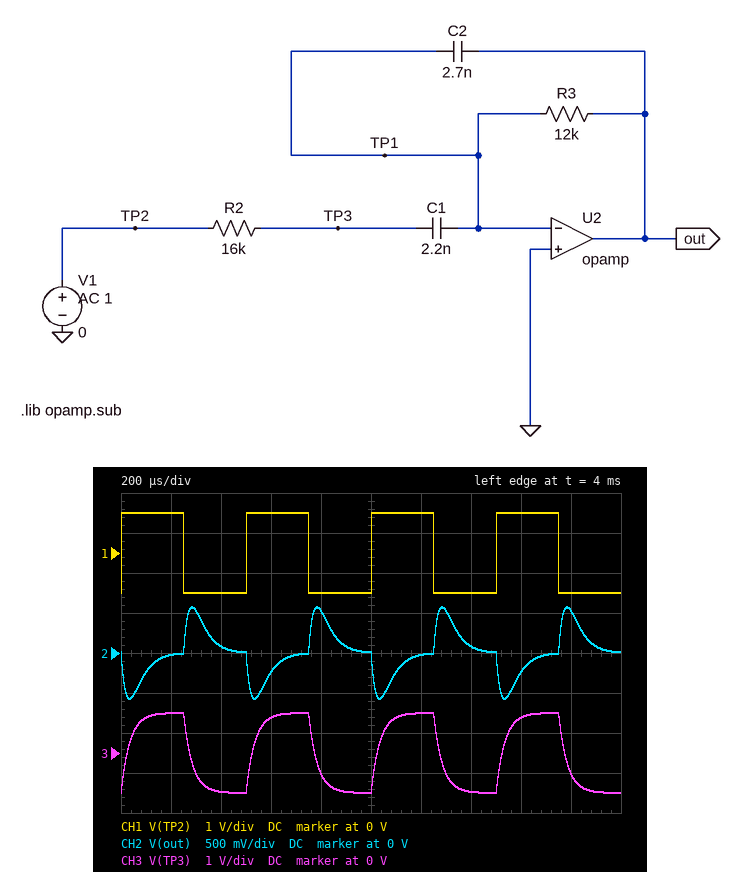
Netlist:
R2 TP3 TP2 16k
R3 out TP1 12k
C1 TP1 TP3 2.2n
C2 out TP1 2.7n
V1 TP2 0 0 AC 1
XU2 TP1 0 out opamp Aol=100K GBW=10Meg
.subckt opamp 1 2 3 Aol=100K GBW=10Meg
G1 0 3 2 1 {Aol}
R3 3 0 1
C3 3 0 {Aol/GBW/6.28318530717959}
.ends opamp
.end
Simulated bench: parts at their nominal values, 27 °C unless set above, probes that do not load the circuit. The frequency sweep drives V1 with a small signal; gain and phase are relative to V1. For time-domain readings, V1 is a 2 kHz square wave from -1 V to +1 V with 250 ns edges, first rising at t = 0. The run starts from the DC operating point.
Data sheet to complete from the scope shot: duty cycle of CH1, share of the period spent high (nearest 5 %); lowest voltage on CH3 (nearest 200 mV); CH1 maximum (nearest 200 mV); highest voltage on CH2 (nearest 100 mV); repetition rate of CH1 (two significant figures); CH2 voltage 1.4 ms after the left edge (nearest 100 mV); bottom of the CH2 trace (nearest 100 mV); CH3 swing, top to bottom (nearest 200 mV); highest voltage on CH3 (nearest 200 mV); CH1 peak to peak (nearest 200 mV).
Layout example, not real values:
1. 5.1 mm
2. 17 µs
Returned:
1. 50 %
2. -1.0 V
3. 1.0 V
4. 600 mV
5. 2.0 kHz
6. 100 mV
7. -600 mV
8. 2.0 V
9. 1.0 V
10. 2.0 V
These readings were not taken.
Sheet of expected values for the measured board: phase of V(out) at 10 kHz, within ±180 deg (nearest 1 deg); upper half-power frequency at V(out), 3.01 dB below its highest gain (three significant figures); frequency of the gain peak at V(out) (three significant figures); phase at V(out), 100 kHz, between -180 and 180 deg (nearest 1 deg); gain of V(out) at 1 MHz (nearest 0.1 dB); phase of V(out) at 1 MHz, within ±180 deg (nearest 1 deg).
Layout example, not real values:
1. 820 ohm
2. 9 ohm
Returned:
1. 140 deg
2. 11.4 kHz
3. 4.71 kHz
4. 95 deg
5. -48.7 dB
6. 85 deg
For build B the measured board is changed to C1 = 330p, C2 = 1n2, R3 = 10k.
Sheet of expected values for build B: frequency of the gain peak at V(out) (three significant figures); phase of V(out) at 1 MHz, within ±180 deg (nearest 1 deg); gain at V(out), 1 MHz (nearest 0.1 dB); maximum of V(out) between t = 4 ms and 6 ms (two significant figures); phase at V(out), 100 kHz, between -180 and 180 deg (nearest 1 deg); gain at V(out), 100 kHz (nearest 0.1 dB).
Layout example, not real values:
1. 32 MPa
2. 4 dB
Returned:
1. 20.0 kHz
2. 87 deg
3. -41.7 dB
4. 290 mV
5. 114 deg
6. -22.1 dB
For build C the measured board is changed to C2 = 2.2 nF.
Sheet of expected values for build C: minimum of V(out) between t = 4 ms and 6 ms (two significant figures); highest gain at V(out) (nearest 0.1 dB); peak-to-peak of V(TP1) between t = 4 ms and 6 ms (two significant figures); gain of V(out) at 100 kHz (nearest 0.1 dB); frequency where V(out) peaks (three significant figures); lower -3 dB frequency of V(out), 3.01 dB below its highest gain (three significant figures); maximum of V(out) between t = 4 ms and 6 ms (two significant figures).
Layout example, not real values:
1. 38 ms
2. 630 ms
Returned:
1. -630 mV
2. -7.4 dB
3. 1.8 mV
4. -26.9 dB
5. 5.22 kHz
6. 2.15 kHz
7. 630 mV
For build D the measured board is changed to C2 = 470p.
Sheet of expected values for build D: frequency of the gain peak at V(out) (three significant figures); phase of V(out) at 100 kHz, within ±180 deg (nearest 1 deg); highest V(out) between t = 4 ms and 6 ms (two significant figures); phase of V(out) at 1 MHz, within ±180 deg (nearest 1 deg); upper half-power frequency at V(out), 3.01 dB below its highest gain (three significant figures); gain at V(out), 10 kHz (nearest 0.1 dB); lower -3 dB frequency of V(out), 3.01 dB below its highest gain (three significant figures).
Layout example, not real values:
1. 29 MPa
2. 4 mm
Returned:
1. 11.3 kHz
2. 108 deg
3. 1.1 V
4. 86 deg
5. 36.2 kHz
6. -3.8 dB
7. 3.52 kHz
